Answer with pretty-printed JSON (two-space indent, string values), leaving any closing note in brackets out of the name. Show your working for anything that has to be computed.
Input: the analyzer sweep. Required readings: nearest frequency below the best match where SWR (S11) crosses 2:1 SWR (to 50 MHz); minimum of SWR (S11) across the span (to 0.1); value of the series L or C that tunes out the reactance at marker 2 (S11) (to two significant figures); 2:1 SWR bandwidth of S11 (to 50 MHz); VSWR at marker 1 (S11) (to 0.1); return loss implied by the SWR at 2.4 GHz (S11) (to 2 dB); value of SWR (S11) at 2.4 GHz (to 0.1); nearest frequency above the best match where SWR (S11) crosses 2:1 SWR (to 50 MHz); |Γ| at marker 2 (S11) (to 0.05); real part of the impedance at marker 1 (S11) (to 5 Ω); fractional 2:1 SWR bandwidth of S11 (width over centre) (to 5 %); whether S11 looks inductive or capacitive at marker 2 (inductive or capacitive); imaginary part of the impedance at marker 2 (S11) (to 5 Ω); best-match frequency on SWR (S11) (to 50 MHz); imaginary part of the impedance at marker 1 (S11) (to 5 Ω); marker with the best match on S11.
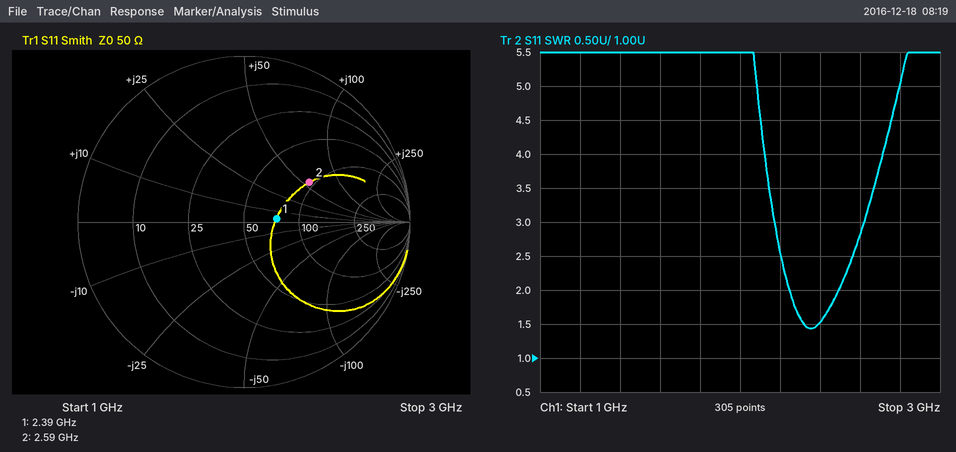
{
  "nearest frequency below the best match where SWR (S11) crosses 2:1 SWR": "2.25 GHz",
  "minimum of SWR (S11) across the span": "1.4",
  "value of the series L or C that tunes out the reactance at marker 2 (S11)": "C = 1/(2π × 2.59 GHz × 55 Ω) ≈ 1.1 pF",
  "2:1 SWR bandwidth of S11": "2.50 GHz − 2.25 GHz = 250 MHz",
  "VSWR at marker 1 (S11)": "1.5",
  "return loss implied by the SWR at 2.4 GHz (S11)": "−20 log10((1.5 − 1)/(1.5 + 1)) ≈ 14 dB",
  "value of SWR (S11) at 2.4 GHz": "1.5",
  "nearest frequency above the best match where SWR (S11) crosses 2:1 SWR": "2.50 GHz",
  "|Γ| at marker 2 (S11)": "0.45",
  "real part of the impedance at marker 1 (S11)": "75 Ω",
  "fractional 2:1 SWR bandwidth of S11 (width over centre)": "250 MHz / 2.375 GHz ≈ 10 %",
  "whether S11 looks inductive or capacitive at marker 2": "inductive",
  "imaginary part of the impedance at marker 2 (S11)": "+55 Ω",
  "best-match frequency on SWR (S11)": "2.35 GHz",
  "imaginary part of the impedance at marker 1 (S11)": "+5 Ω",
  "marker with the best match on S11": "marker 1"
}
